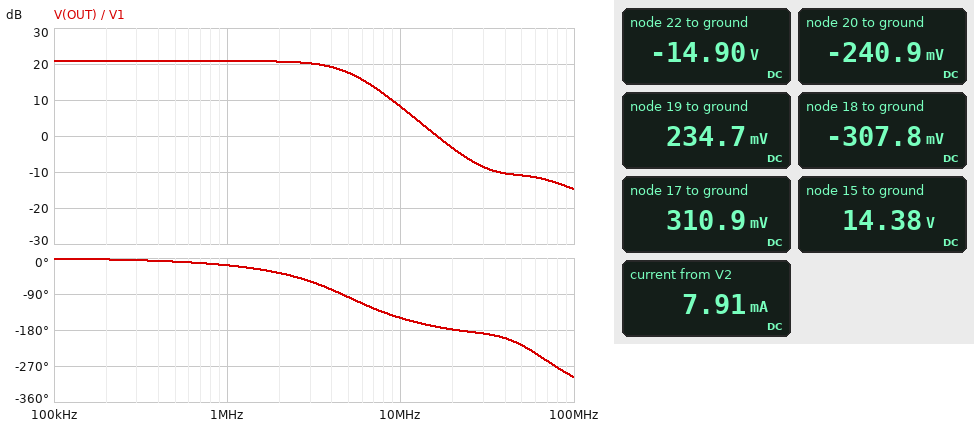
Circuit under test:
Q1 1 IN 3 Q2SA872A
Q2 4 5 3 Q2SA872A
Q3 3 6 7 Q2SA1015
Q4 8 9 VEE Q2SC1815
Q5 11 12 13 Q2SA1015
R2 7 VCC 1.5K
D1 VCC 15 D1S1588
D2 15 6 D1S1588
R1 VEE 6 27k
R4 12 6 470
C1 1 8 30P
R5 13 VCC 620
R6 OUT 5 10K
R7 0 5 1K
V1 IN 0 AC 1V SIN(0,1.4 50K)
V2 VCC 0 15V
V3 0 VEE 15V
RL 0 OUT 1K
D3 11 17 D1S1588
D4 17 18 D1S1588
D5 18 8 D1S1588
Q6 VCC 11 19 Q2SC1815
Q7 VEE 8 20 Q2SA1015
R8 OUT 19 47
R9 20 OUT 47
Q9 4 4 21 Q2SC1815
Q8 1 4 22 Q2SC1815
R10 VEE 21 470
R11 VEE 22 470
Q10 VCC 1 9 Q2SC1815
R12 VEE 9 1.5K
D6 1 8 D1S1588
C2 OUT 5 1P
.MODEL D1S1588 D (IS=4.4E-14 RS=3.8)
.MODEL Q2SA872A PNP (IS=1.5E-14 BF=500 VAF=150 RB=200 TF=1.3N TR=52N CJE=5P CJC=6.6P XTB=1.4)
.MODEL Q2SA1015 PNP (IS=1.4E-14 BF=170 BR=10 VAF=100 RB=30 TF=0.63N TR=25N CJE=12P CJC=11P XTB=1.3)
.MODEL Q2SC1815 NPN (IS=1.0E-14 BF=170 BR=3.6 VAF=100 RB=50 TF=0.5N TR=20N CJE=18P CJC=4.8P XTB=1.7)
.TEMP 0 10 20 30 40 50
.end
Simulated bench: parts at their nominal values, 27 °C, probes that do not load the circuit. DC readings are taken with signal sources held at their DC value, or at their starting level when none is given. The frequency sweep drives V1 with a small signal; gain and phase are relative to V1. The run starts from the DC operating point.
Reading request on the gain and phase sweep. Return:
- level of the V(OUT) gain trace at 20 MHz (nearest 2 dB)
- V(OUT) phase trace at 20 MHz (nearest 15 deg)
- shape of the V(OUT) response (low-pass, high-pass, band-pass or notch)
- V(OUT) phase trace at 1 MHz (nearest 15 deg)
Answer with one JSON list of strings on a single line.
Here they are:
["-4 dB", "-180 deg", "low-pass", "-15 deg"]
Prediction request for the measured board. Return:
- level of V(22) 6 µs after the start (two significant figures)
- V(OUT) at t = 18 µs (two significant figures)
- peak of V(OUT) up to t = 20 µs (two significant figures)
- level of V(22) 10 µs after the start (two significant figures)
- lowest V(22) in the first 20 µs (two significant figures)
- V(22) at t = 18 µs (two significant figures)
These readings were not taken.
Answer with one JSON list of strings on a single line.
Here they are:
["-15 V", "-9.3 V", "13 V", "-15 V", "-15 V", "-15 V"]
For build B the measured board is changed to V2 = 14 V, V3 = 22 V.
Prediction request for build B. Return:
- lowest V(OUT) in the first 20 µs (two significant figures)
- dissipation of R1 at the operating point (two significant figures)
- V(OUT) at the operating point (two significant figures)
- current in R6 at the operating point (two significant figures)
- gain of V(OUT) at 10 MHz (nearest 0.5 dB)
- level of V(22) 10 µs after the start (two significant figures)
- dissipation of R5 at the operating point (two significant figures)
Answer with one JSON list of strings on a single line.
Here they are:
["-15 V", "45 mW", "-3.1 mV", "320 nA", "8.5 dB", "-22 V", "600 µW"]
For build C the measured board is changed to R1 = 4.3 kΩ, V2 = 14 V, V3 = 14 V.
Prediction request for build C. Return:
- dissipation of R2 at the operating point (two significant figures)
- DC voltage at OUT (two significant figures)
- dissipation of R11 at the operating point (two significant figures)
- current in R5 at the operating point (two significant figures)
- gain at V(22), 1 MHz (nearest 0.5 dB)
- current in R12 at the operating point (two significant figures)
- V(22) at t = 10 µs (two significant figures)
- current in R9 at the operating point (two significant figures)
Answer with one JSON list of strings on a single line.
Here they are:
["370 µW", "-4.3 mV", "29 µW", "1.2 mA", "-6.0 dB", "440 µA", "-14 V", "5.2 mA"]
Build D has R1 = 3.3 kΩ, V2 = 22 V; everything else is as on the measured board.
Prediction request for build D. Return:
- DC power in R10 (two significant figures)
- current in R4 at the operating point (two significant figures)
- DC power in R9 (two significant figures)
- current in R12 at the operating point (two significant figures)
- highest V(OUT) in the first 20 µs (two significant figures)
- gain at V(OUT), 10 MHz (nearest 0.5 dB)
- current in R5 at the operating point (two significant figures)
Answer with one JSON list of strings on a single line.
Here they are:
["34 µW", "6.2 µA", "1.3 mW", "440 µA", "15 V", "10.0 dB", "1.3 mA"]
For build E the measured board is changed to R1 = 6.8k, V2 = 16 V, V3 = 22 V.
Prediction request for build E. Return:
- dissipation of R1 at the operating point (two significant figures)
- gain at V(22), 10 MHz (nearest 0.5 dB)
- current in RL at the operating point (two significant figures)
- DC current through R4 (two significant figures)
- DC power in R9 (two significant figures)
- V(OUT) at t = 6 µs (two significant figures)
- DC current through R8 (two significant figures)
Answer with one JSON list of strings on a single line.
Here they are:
["200 mW", "2.5 dB", "4.2 µA", "5.9 µA", "1.3 mW", "14 V", "5.2 mA"]
